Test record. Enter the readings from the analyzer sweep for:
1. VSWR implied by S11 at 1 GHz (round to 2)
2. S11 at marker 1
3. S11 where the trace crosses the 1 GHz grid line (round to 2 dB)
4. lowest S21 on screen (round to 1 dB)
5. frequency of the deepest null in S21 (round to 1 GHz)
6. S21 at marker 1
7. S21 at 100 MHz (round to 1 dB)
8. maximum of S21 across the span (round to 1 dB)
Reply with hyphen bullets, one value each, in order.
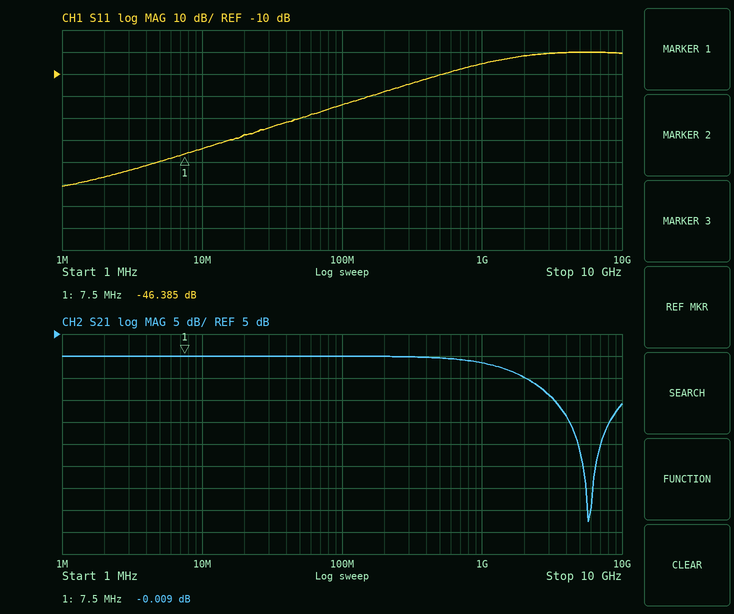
- 4
- -46.385 dB
- -6 dB
- -38 dB
- 6 GHz
- -0.009 dB
- 0 dB
- 0 dB
